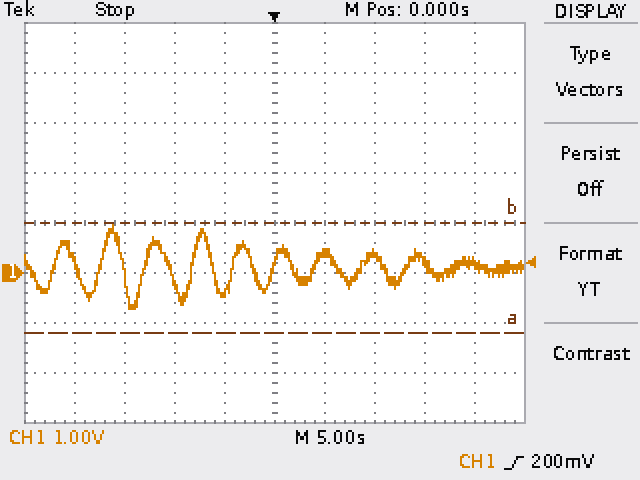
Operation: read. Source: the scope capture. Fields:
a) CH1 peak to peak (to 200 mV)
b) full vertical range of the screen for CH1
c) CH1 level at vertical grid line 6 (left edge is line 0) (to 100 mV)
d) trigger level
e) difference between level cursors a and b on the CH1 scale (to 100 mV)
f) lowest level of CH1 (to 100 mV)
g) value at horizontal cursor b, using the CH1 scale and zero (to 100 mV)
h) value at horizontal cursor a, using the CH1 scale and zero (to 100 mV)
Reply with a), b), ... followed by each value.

a) 1.6 V
b) 8 V
c) 400 mV
d) 200 mV
e) 2.2 V
f) -700 mV
g) 1.0 V
h) -1.2 V
